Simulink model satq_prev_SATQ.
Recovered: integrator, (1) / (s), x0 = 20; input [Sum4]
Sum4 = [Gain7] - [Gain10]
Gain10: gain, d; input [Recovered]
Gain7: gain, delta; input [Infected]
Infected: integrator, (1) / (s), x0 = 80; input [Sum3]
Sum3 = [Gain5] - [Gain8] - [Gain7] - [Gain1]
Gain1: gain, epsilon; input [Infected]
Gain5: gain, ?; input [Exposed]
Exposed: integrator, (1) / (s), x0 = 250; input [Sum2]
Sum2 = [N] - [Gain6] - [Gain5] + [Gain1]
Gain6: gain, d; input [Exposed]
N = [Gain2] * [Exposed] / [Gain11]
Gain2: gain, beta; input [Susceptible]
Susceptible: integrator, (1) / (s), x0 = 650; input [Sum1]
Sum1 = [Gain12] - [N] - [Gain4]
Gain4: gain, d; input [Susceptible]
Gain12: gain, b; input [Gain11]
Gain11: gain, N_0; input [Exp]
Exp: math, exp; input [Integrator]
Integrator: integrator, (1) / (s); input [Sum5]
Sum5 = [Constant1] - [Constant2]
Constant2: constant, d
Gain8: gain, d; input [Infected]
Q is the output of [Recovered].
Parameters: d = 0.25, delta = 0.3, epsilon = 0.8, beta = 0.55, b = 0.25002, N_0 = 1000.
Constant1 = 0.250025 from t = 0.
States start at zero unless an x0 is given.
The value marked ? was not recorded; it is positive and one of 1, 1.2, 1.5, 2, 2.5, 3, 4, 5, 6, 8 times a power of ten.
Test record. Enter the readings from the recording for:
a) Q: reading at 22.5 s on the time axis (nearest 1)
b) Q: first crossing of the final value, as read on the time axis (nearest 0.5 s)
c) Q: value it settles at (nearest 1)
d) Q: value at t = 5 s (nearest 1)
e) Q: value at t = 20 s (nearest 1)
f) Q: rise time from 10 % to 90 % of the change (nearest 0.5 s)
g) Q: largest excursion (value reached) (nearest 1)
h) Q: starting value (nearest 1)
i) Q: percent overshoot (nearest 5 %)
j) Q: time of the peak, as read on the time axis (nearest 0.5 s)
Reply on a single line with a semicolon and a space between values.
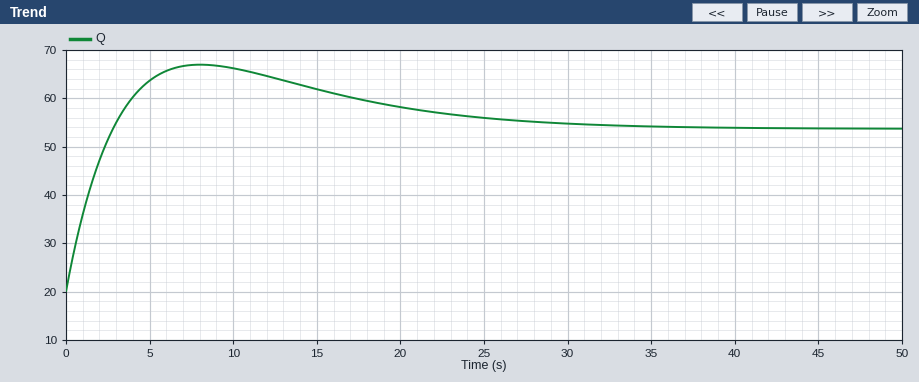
57; 3.0 s; 54; 64; 58; 2.0 s; 67; 20; 40 %; 8.0 s
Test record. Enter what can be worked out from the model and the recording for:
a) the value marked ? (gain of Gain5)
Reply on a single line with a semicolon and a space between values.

0.4
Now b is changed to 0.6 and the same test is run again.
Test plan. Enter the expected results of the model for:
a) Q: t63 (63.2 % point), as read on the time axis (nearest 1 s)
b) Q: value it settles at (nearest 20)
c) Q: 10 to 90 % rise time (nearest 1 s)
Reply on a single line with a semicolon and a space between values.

10 s; 360; 13 s
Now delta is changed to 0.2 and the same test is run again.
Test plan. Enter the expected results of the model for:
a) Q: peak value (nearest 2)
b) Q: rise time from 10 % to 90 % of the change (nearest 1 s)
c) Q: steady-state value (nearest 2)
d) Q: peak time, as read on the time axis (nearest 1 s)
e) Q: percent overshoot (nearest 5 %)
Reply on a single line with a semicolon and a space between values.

52; 3 s; 46; 9 s; 20 %
